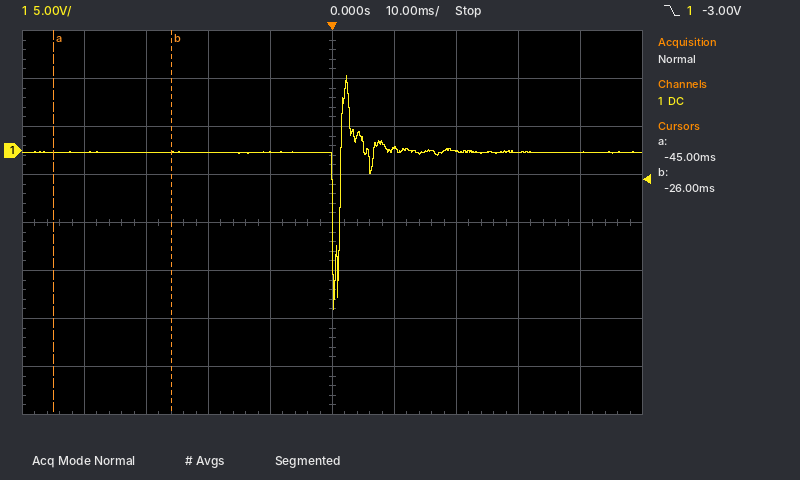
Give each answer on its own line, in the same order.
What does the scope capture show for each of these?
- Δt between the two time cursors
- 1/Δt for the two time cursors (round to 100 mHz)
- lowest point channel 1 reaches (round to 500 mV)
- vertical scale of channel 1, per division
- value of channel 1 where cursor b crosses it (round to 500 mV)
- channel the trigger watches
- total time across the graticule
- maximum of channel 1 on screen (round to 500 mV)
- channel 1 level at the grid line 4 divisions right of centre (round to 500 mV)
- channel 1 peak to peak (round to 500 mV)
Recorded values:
19 ms
52.6 Hz
-16.5 V
5 V
0.0 V
channel 1
100 ms
8.0 V
0.0 V
24.5 V
